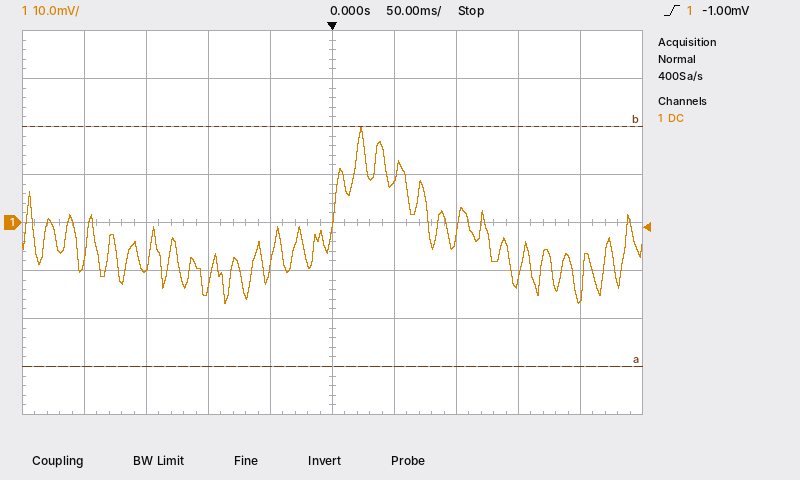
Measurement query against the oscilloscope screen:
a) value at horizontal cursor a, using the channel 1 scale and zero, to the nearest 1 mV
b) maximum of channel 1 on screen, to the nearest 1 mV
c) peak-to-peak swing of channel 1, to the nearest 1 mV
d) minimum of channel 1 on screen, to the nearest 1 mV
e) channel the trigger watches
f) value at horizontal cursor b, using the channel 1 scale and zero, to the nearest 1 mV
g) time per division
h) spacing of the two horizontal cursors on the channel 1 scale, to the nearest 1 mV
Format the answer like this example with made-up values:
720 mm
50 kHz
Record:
-30 mV
20 mV
37 mV
-17 mV
channel 1
20 mV
50 ms
50 mV
